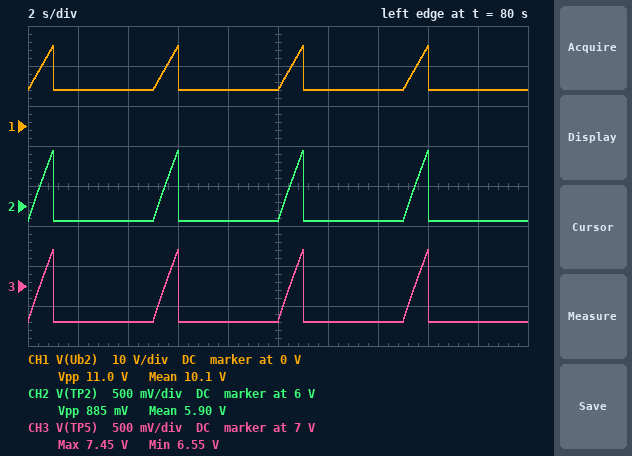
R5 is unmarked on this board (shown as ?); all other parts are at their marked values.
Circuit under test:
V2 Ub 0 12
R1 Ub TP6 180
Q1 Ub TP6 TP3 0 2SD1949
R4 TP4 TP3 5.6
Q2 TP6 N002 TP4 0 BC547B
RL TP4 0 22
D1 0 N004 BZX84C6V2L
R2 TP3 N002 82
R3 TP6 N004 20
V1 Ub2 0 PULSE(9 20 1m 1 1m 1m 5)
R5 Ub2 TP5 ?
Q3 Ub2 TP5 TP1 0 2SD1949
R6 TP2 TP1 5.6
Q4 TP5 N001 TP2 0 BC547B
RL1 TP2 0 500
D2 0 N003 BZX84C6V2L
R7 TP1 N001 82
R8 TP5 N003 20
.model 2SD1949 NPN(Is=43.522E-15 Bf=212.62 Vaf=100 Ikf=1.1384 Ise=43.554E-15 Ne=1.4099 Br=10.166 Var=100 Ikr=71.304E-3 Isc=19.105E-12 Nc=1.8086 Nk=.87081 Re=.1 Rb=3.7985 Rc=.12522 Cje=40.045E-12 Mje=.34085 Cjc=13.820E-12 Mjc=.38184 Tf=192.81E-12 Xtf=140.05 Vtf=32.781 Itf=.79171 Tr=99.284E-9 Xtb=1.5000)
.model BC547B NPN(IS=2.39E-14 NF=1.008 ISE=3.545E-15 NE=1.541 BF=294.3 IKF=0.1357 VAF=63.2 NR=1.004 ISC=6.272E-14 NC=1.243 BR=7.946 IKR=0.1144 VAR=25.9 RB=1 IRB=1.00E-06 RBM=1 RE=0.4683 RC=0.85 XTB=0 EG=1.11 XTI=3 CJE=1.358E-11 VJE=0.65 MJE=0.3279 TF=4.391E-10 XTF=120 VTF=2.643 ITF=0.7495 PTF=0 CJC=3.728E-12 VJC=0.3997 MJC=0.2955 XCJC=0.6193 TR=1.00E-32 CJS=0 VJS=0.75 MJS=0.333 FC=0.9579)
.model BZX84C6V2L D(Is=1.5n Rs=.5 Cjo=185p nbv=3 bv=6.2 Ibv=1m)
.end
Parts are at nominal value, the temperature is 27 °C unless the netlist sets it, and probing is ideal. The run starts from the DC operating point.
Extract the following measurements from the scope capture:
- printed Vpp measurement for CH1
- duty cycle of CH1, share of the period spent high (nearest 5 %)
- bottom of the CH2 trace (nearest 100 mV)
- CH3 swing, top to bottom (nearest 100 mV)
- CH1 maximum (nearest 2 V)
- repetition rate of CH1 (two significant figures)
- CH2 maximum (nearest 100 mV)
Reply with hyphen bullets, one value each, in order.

- 11.0 V
- 10 %
- 5.8 V
- 900 mV
- 20 V
- 200 mHz
- 6.7 V
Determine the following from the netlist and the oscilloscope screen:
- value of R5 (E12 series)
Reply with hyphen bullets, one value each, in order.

- 270 Ω
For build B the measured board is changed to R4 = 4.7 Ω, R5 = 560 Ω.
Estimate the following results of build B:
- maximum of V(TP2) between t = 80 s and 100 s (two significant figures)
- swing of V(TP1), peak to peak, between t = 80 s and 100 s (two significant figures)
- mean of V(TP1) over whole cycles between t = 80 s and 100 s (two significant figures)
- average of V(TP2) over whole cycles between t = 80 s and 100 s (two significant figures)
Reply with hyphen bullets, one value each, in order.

- 6.2 V
- 510 mV
- 5.8 V
- 5.7 V
